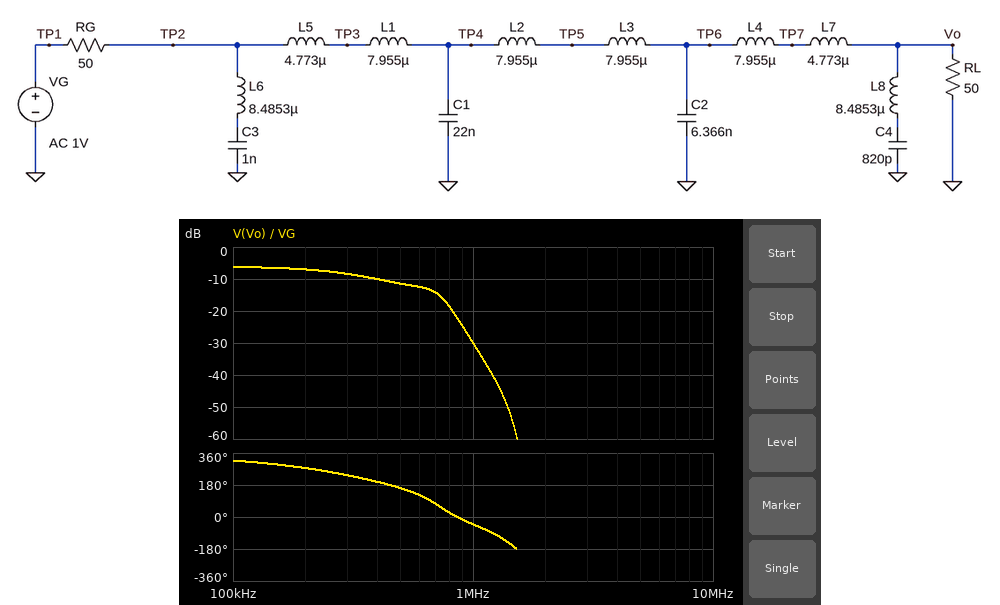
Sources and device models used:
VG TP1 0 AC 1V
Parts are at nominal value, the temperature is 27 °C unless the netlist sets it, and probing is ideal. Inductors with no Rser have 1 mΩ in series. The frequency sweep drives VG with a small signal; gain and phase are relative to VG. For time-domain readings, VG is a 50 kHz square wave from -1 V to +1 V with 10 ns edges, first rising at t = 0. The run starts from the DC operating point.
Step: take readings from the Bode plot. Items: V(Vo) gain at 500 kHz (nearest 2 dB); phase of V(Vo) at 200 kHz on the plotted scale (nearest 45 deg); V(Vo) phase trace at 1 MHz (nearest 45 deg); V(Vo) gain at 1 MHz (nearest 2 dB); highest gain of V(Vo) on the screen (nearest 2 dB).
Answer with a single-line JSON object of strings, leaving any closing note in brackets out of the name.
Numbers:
{"V(Vo) gain at 500 kHz": "-12 dB", "phase of V(Vo) at 200 kHz on the plotted scale": "270 deg", "V(Vo) phase trace at 1 MHz": "-45 deg", "V(Vo) gain at 1 MHz": "-30 dB", "highest gain of V(Vo) on the screen": "-6 dB"}
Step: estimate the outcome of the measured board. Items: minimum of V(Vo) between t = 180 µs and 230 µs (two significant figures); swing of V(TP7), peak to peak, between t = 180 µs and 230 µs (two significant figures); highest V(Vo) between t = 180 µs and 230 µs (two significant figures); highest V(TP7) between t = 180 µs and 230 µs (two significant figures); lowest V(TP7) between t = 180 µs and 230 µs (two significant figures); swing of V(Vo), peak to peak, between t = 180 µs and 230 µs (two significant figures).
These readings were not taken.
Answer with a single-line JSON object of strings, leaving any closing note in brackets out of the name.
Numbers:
{"minimum of V(Vo) between t = 180 µs and 230 µs": "-520 mV", "swing of V(TP7), peak to peak, between t = 180 µs and 230 µs": "1.0 V", "highest V(Vo) between t = 180 µs and 230 µs": "520 mV", "highest V(TP7) between t = 180 µs and 230 µs": "520 mV", "lowest V(TP7) between t = 180 µs and 230 µs": "-520 mV", "swing of V(Vo), peak to peak, between t = 180 µs and 230 µs": "1.0 V"}
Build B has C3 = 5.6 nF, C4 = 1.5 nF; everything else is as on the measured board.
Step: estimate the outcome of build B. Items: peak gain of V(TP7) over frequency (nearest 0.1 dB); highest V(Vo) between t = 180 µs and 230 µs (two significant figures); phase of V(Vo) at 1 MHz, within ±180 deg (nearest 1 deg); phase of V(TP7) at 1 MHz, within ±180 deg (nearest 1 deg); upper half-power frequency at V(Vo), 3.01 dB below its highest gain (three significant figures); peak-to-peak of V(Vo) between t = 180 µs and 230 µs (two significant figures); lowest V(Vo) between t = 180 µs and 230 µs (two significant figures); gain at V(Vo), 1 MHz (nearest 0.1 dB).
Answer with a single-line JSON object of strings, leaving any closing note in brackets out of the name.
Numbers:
{"peak gain of V(TP7) over frequency": "-6.0 dB", "highest V(Vo) between t = 180 µs and 230 µs": "560 mV", "phase of V(Vo) at 1 MHz, within ±180 deg": "-12 deg", "phase of V(TP7) at 1 MHz, within ±180 deg": "42 deg", "upper half-power frequency at V(Vo), 3.01 dB below its highest gain": "548 kHz", "peak-to-peak of V(Vo) between t = 180 µs and 230 µs": "1.1 V", "lowest V(Vo) between t = 180 µs and 230 µs": "-560 mV", "gain at V(Vo), 1 MHz": "-37.1 dB"}
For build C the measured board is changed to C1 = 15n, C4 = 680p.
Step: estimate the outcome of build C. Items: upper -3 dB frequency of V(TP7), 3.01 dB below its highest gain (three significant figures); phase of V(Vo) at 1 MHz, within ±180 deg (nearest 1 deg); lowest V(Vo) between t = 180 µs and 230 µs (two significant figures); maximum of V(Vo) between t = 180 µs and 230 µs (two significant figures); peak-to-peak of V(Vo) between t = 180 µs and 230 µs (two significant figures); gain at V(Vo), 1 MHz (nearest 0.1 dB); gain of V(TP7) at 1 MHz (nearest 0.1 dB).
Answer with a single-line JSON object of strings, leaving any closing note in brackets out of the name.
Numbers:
{"upper -3 dB frequency of V(TP7), 3.01 dB below its highest gain": "560 kHz", "phase of V(Vo) at 1 MHz, within ±180 deg": "-35 deg", "lowest V(Vo) between t = 180 µs and 230 µs": "-550 mV", "maximum of V(Vo) between t = 180 µs and 230 µs": "550 mV", "peak-to-peak of V(Vo) between t = 180 µs and 230 µs": "1.1 V", "gain at V(Vo), 1 MHz": "-26.0 dB", "gain of V(TP7) at 1 MHz": "-25.8 dB"}
